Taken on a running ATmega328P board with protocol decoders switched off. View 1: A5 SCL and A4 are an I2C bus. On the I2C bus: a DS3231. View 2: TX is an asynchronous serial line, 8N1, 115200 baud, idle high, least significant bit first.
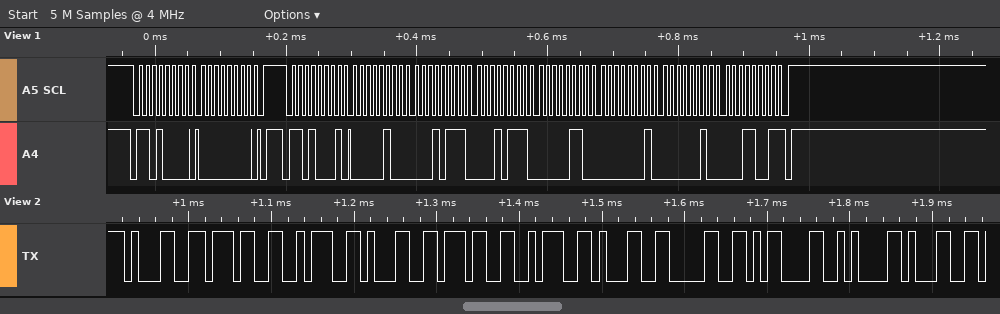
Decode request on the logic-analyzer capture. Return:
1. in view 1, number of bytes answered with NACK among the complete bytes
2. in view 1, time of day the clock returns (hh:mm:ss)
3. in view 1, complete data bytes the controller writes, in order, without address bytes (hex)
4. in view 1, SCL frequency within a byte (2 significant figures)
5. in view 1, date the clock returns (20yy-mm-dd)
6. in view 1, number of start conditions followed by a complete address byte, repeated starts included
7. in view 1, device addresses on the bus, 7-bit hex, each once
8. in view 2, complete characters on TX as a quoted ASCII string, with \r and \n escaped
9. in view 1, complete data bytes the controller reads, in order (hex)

1
17:17:04
00
100 kHz
2019-02-01
2
0x68
"17:17:10\r\n1"
04 17 17 06 01 02 19
